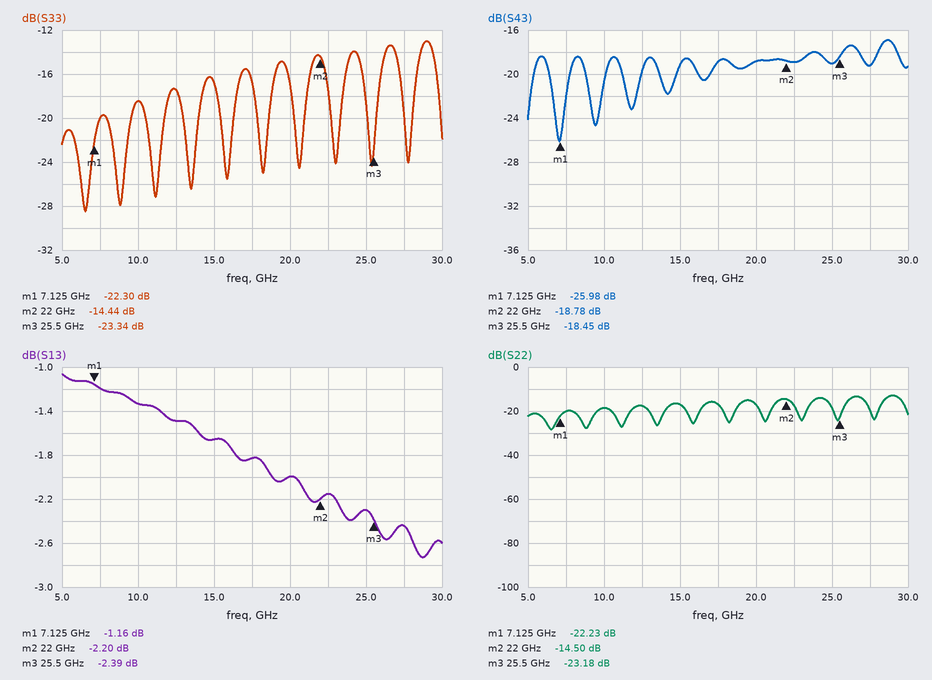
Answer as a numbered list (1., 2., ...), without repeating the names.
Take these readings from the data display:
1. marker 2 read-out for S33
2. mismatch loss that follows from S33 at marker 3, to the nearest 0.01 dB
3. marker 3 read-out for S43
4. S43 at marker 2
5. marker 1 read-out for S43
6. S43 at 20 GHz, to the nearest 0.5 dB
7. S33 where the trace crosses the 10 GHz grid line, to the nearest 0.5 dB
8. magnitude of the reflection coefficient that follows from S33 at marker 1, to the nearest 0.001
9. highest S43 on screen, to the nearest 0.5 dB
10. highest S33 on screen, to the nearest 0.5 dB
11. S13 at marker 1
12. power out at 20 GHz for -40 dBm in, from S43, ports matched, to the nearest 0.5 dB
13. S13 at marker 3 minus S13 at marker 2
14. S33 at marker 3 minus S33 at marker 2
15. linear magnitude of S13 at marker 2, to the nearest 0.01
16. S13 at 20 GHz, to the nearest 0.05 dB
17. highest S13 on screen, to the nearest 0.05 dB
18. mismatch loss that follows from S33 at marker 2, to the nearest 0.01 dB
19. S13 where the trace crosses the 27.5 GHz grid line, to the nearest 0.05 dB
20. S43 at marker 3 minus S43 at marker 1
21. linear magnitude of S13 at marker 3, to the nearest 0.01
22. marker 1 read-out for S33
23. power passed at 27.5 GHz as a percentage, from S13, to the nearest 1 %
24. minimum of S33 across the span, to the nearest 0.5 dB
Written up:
1. -14.44 dB
2. 0.02 dB
3. -18.45 dB
4. -18.78 dB
5. -25.98 dB
6. -19.0 dB
7. -18.5 dB
8. 0.077
9. -17.0 dB
10. -13.0 dB
11. -1.16 dB
12. -59.0 dBm
13. -0.19 dB
14. -8.90 dB
15. 0.78
16. -2.00 dB
17. -1.05 dB
18. 0.16 dB
19. -2.45 dB
20. 7.53 dB
21. 0.76
22. -22.30 dB
23. 57 %
24. -28.5 dB
